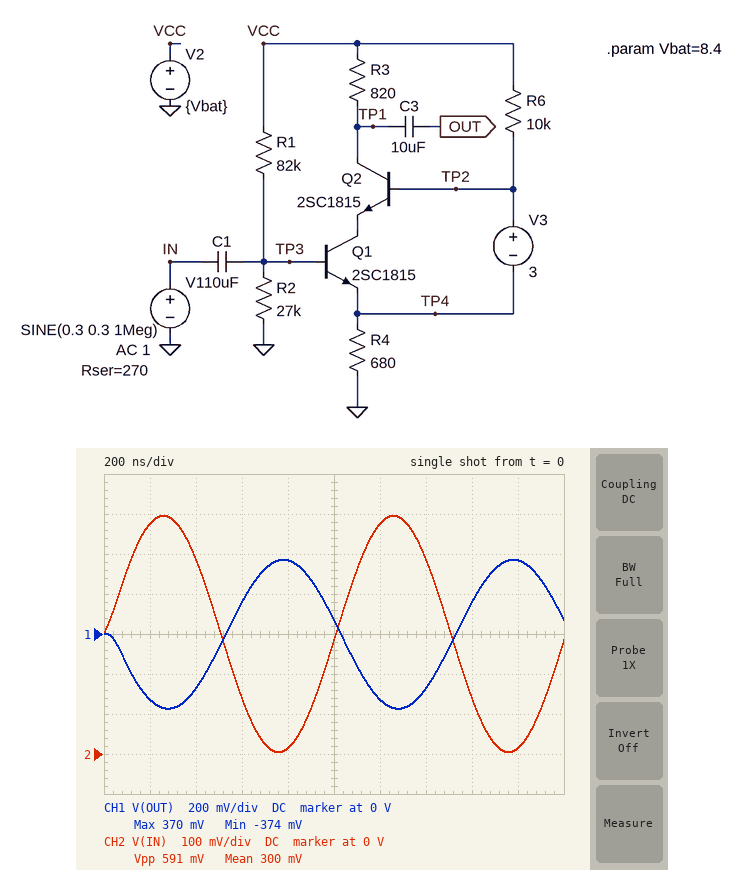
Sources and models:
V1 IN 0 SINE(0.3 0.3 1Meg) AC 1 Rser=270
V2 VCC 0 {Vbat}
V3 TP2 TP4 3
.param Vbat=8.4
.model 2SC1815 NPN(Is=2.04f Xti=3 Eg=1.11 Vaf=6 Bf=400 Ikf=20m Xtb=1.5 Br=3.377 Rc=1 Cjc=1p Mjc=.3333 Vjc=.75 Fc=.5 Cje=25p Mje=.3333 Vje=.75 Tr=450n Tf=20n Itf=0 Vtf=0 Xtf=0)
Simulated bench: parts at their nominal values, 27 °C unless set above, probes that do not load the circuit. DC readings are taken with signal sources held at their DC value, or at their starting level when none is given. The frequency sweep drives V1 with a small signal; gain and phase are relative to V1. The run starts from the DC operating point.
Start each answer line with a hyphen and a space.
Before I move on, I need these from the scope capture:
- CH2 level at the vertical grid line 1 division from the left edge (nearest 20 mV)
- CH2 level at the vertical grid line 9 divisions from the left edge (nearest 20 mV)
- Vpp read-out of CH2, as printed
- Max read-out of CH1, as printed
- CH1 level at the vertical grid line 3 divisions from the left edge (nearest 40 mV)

- 580 mV
- 20 mV
- 591 mV
- 370 mV
- 160 mV
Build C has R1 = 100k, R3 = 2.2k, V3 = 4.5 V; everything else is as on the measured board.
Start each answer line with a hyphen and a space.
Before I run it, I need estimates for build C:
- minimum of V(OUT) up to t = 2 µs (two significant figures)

- -820 mV
